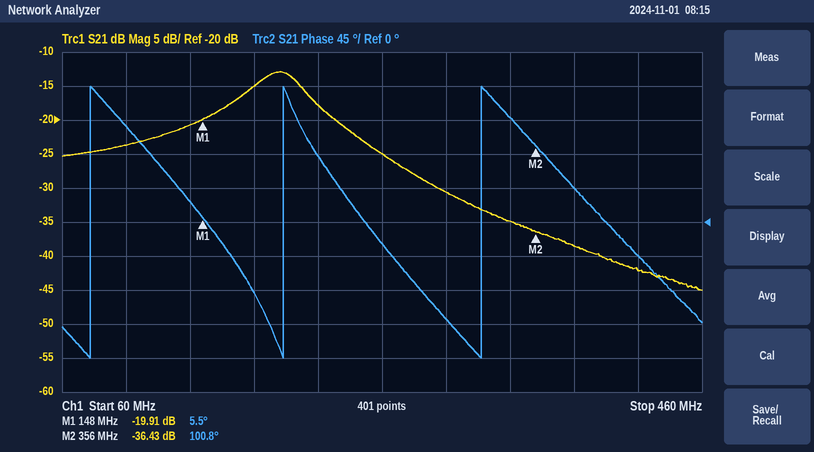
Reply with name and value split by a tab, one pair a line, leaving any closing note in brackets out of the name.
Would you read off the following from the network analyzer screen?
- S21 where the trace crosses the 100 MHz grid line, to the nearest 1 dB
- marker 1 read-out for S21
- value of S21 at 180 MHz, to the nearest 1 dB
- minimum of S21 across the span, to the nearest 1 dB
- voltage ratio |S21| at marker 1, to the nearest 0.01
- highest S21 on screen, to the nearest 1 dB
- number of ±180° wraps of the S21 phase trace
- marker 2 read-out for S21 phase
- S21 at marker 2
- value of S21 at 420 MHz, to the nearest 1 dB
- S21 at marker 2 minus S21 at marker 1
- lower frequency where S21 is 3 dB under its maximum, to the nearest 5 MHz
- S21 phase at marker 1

S21 where the trace crosses the 100 MHz grid line, to the nearest 1 dB	-24 dB
marker 1 read-out for S21	-19.91 dB
value of S21 at 180 MHz, to the nearest 1 dB	-15 dB
minimum of S21 across the span, to the nearest 1 dB	-45 dB
voltage ratio |S21| at marker 1, to the nearest 0.01	0.10
highest S21 on screen, to the nearest 1 dB	-13 dB
number of ±180° wraps of the S21 phase trace	3
marker 2 read-out for S21 phase	100.8°
S21 at marker 2	-36.43 dB
value of S21 at 420 MHz, to the nearest 1 dB	-42 dB
S21 at marker 2 minus S21 at marker 1	-16.52 dB
lower frequency where S21 is 3 dB under its maximum, to the nearest 5 MHz	175 MHz
S21 phase at marker 1	5.5°
